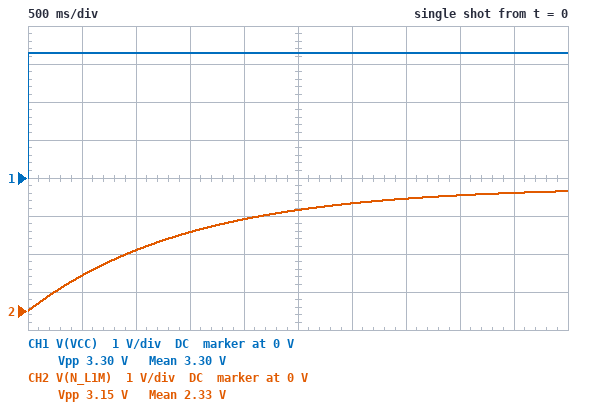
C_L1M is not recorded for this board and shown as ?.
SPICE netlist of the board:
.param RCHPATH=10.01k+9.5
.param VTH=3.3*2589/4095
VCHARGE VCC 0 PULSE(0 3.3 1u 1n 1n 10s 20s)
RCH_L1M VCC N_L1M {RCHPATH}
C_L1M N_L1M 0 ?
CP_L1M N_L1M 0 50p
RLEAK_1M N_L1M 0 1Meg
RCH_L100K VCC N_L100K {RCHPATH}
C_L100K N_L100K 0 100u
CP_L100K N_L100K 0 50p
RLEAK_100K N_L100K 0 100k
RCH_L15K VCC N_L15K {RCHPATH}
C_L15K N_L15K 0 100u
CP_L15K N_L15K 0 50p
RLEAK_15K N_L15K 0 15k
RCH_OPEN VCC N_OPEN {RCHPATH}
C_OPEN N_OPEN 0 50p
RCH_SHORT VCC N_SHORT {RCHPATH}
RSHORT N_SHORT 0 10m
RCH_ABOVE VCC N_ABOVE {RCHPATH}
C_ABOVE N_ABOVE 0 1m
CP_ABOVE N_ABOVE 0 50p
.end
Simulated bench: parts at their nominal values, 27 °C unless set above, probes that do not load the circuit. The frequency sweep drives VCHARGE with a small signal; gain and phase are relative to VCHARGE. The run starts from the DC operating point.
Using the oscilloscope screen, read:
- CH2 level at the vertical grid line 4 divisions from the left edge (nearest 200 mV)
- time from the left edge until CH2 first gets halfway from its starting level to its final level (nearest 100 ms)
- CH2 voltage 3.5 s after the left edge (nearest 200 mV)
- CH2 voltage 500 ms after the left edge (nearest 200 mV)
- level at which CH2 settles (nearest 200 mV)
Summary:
2.4 V
1.0 s
3.0 V
1.0 V
3.2 V
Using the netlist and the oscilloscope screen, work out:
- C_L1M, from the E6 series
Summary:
150 µF
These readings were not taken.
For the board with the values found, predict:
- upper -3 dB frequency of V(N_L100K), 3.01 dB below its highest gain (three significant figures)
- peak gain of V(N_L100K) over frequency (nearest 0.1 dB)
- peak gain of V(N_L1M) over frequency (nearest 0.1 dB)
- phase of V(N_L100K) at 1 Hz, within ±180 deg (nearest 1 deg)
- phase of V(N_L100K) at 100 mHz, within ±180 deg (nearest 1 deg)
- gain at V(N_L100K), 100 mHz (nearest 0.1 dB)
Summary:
175 mHz
-0.8 dB
-0.1 dB
-80 deg
-30 deg
-2.1 dB
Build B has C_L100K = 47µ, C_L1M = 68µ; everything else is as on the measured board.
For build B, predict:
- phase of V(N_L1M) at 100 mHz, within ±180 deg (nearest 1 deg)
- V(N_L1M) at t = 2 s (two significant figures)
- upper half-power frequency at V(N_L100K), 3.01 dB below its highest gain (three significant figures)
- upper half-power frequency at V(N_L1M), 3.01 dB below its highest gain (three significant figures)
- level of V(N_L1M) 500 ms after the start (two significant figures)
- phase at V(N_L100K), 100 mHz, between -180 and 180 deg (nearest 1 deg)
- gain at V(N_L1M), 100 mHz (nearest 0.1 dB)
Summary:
-23 deg
3.1 V
372 mHz
236 mHz
1.7 V
-15 deg
-0.8 dB
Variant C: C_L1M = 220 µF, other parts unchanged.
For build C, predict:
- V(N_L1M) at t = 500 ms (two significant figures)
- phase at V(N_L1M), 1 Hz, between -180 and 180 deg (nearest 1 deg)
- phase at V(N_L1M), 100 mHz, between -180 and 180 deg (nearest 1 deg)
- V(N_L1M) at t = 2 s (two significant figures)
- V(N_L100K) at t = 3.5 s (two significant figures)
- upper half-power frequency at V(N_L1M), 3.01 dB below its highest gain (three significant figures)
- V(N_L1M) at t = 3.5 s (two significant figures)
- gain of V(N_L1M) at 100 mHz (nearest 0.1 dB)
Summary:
670 mV
-86 deg
-54 deg
2.0 V
2.9 V
72.9 mHz
2.6 V
-4.7 dB
